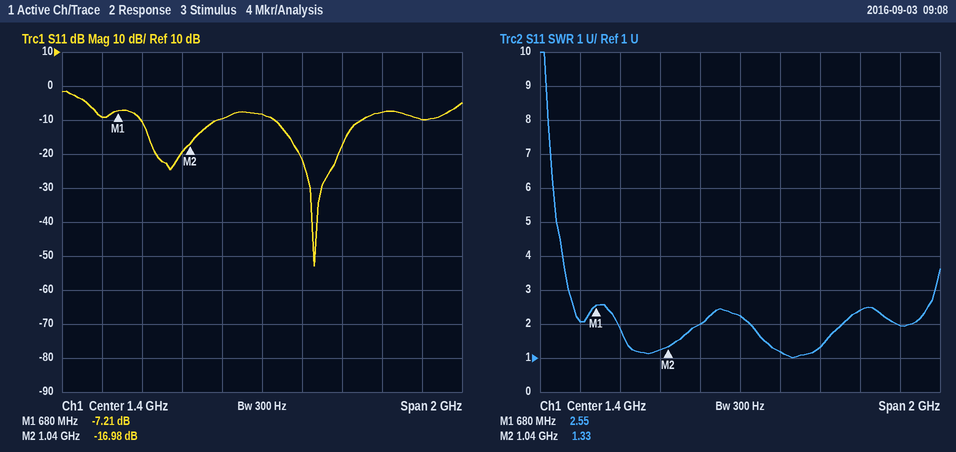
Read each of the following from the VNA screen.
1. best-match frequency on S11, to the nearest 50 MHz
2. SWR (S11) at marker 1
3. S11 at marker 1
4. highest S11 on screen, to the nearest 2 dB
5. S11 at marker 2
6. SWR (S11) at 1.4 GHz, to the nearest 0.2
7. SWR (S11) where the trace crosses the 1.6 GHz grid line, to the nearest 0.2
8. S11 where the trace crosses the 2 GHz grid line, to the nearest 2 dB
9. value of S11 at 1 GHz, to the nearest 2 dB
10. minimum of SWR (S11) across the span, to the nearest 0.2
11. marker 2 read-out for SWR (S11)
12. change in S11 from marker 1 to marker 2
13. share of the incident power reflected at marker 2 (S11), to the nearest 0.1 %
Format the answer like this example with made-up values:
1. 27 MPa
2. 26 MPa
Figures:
1. 1.65 GHz
2. 2.55
3. -7.21 dB
4. -2 dB
5. -16.98 dB
6. 2.2
7. 1.2
8. -8 dB
9. -20 dB
10. 1.0
11. 1.33
12. -9.77 dB
13. 2.0 %
